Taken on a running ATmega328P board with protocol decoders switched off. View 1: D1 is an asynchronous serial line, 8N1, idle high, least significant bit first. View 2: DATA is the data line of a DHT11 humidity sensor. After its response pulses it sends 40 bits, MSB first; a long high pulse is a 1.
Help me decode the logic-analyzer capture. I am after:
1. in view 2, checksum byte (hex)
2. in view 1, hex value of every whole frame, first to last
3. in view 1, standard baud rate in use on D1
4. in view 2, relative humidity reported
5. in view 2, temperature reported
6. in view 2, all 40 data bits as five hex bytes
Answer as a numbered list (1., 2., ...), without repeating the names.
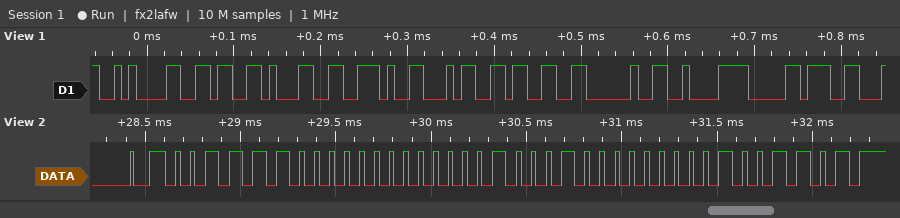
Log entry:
1. 0x4D
2. 0A 36 31 2E 34 33 20 C2 B0
3. 115200 baud
4. 60 %
5. 17.0 °C
6. 3C 00 11 00 4D
